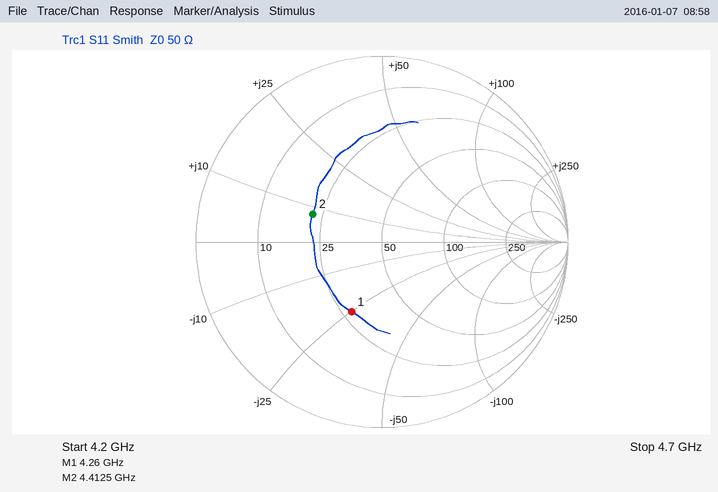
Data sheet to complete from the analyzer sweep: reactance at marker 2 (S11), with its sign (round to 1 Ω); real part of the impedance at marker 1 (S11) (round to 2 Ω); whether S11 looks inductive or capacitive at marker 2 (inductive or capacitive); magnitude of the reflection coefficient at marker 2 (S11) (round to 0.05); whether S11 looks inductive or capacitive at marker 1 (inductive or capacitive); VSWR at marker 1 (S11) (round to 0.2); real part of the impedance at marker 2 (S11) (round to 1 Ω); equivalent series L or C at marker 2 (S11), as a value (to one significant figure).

+8 Ω
28 Ω
inductive
0.40
capacitive
2.4
22 Ω
300 pH
